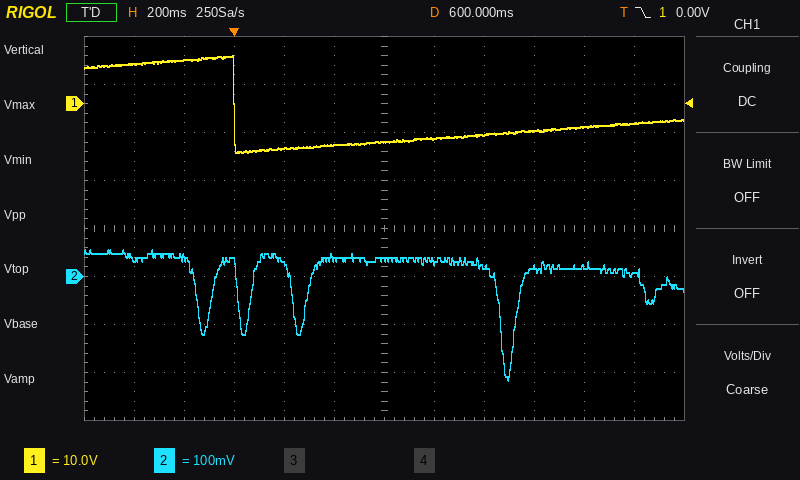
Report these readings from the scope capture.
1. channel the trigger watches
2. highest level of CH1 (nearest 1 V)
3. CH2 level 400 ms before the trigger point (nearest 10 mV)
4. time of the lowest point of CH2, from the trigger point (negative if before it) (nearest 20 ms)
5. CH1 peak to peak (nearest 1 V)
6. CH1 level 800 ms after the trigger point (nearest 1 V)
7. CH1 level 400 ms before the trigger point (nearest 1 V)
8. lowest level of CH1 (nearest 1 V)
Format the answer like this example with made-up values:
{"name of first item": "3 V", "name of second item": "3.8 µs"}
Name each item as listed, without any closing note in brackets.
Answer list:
{"channel the trigger watches": "CH1", "highest level of CH1": "10 V", "CH2 level 400 ms before the trigger point": "40 mV", "time of the lowest point of CH2, from the trigger point (negative if before it)": "+1.10 s", "CH1 peak to peak": "20 V", "CH1 level 800 ms after the trigger point": "-7 V", "CH1 level 400 ms before the trigger point": "8 V", "lowest level of CH1": "-10 V"}
